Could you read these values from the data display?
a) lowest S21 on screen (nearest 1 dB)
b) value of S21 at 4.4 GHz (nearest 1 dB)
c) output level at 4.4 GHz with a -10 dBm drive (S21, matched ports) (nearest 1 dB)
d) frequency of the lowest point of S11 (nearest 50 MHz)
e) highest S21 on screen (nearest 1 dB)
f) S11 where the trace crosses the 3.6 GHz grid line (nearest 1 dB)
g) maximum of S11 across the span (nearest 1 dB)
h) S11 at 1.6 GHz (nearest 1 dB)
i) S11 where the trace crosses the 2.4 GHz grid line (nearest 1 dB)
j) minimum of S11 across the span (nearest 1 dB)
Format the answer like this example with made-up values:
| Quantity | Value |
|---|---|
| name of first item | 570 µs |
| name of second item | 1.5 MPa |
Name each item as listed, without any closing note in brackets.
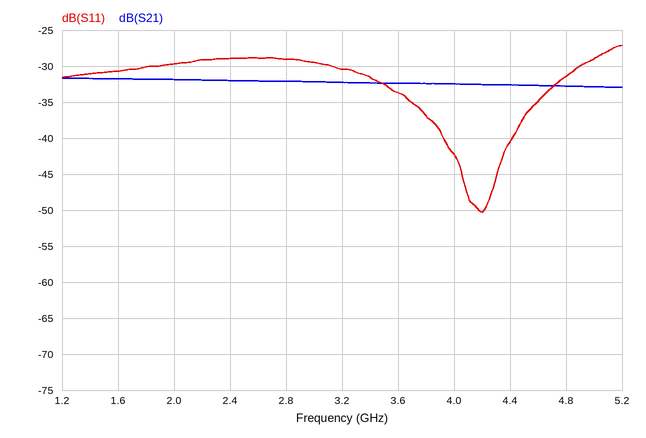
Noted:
| Quantity | Value |
|---|---|
| lowest S21 on screen | -33 dB |
| value of S21 at 4.4 GHz | -33 dB |
| output level at 4.4 GHz with a -10 dBm drive (S21, matched ports) | -43 dBm |
| frequency of the lowest point of S11 | 4.20 GHz |
| highest S21 on screen | -32 dB |
| S11 where the trace crosses the 3.6 GHz grid line | -34 dB |
| maximum of S11 across the span | -27 dB |
| S11 at 1.6 GHz | -31 dB |
| S11 where the trace crosses the 2.4 GHz grid line | -29 dB |
| minimum of S11 across the span | -50 dB |
